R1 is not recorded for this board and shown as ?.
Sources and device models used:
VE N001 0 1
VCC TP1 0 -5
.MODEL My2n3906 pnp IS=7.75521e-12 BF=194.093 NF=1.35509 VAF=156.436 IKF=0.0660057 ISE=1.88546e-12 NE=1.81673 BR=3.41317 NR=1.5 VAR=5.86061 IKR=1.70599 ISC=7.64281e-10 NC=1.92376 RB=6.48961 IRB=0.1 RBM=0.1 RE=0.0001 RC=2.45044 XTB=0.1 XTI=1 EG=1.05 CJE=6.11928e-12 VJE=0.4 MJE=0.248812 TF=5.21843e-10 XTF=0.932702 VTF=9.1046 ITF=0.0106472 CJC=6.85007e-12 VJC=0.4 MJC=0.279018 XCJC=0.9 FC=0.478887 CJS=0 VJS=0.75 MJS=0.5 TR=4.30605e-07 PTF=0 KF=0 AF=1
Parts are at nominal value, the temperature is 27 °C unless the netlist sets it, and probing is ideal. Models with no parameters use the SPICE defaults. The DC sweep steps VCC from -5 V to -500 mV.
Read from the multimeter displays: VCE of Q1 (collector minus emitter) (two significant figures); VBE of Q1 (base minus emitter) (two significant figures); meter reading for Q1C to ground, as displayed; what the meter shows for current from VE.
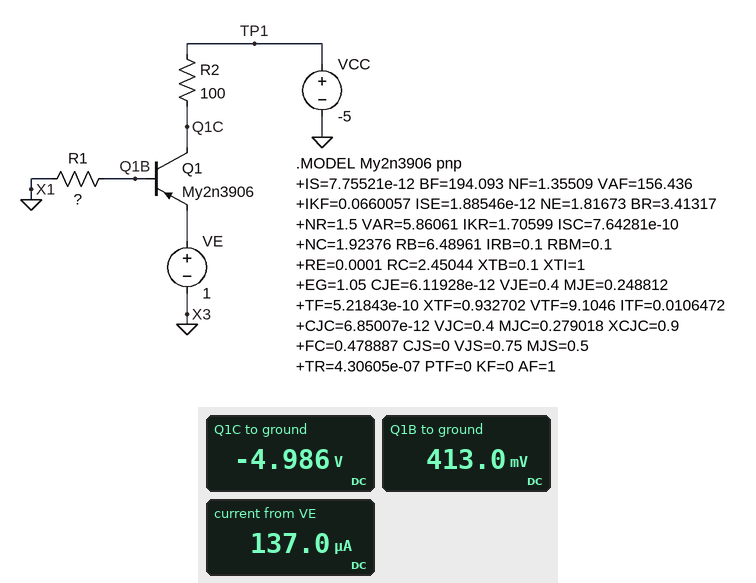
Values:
-6.0 V
-590 mV
-4.986 V
137.0 µA
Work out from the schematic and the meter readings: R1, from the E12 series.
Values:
330 kΩ
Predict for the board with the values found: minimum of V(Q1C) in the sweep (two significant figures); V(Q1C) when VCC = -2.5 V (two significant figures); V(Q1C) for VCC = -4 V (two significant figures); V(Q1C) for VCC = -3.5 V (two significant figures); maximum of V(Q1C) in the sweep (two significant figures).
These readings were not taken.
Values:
-5.0 V
-2.5 V
-4.0 V
-3.5 V
-490 mV
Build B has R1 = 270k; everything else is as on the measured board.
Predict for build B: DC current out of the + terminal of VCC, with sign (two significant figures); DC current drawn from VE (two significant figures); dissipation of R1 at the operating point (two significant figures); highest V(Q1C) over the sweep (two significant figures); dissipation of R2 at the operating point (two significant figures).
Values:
-170 µA
170 µA
610 nW
-480 mV
2.8 µW
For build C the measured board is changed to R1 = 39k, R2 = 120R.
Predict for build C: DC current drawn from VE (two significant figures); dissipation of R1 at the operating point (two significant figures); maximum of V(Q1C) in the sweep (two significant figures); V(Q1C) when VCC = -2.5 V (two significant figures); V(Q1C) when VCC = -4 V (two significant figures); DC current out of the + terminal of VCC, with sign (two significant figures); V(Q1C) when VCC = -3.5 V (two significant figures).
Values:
1.1 mA
2.9 µW
-370 mV
-2.4 V
-3.9 V
-1.1 mA
-3.4 V
